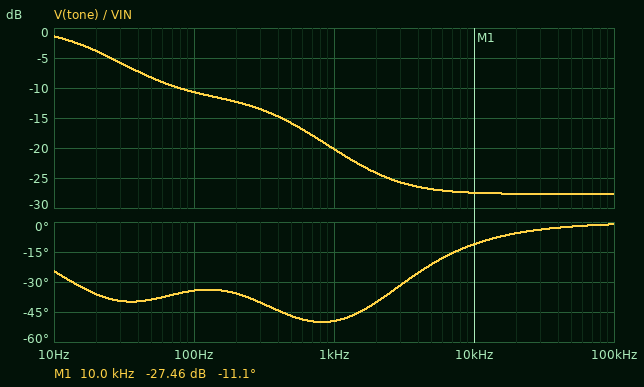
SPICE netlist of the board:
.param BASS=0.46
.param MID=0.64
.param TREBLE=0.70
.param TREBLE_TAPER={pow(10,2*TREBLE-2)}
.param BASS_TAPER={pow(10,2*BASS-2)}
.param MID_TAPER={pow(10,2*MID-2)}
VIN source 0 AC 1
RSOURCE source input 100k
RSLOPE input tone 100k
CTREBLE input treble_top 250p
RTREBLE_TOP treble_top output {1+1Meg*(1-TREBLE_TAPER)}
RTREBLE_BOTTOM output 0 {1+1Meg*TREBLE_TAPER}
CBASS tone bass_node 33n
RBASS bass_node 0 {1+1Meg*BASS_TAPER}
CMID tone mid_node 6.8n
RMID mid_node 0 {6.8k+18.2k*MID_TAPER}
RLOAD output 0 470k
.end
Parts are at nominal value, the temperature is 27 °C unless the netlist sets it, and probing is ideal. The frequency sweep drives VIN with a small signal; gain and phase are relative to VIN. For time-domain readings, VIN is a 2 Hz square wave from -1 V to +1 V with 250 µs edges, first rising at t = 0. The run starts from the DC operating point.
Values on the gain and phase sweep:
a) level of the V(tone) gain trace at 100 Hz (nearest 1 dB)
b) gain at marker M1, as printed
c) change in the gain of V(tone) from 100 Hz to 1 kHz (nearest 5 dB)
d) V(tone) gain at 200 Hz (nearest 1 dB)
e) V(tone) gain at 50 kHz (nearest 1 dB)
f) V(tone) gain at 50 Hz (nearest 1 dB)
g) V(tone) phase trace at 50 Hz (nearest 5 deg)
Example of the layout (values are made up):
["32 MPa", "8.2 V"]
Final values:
["-11 dB", "-27.46 dB", "-10 dB", "-12 dB", "-28 dB", "-8 dB", "-40 deg"]
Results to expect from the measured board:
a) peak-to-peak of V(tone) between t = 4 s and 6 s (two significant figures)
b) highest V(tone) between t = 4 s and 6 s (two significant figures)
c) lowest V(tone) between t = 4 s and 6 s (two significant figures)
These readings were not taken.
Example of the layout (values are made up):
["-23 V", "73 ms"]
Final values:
["2.0 V", "1.0 V", "-1.0 V"]
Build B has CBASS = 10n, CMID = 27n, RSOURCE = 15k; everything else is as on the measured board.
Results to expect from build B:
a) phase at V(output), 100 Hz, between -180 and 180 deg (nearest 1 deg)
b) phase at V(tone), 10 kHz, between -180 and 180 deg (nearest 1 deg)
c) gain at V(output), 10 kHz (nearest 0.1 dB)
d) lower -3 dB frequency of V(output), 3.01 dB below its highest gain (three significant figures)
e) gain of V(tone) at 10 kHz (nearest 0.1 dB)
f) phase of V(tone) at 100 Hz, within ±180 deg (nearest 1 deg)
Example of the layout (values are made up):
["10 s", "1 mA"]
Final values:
["79 deg", "-3 deg", "-16.2 dB", "687 Hz", "-22.8 dB", "-57 deg"]
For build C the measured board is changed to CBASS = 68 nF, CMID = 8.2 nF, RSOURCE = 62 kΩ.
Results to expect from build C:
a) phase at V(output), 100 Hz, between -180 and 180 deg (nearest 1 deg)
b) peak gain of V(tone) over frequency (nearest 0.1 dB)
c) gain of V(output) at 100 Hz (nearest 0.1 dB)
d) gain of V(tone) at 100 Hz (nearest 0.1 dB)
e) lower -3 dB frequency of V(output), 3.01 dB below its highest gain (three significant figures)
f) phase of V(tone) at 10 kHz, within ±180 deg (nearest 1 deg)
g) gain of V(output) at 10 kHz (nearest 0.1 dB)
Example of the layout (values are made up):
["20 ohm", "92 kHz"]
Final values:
["77 deg", "0 dB", "-34.6 dB", "-10.0 dB", "631 Hz", "-9 deg", "-19.2 dB"]
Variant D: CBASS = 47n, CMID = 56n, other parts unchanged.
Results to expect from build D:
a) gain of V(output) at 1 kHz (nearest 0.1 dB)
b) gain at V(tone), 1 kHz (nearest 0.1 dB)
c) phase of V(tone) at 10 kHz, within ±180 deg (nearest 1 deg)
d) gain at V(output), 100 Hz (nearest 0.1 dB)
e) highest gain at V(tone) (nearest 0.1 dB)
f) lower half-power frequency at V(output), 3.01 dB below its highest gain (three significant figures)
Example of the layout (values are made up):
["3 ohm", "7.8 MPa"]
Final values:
["-22.6 dB", "-27.2 dB", "-2 deg", "-37.3 dB", "0 dB", "659 Hz"]
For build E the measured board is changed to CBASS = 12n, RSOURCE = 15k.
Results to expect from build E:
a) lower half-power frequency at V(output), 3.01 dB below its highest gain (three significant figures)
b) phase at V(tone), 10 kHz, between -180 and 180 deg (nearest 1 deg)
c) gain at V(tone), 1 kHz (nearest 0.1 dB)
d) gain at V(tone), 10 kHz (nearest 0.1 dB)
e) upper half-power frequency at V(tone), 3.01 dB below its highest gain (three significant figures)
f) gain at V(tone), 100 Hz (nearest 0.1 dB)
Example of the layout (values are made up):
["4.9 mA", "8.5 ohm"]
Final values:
["673 Hz", "-11 deg", "-15.7 dB", "-22.6 dB", "61.6 Hz", "-5.1 dB"]
